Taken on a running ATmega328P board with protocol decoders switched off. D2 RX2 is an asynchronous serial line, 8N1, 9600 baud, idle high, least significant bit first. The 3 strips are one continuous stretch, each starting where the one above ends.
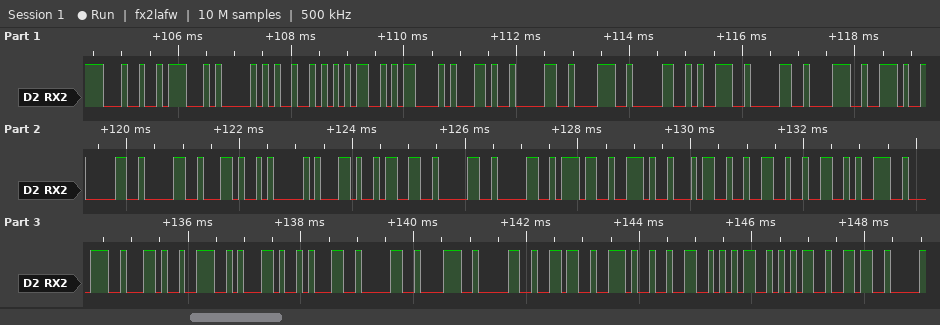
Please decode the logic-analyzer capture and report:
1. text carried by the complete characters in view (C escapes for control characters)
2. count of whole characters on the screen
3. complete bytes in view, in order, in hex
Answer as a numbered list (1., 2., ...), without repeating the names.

1. "$GPRMC,080908.00,A,3007.42298,N,10806.2556"
2. 42
3. 24 47 50 52 4D 43 2C 30 38 30 39 30 38 2E 30 30 2C 41 2C 33 30 30 37 2E 34 32 32 39 38 2C 4E 2C 31 30 38 30 36 2E 32 35 35 36
